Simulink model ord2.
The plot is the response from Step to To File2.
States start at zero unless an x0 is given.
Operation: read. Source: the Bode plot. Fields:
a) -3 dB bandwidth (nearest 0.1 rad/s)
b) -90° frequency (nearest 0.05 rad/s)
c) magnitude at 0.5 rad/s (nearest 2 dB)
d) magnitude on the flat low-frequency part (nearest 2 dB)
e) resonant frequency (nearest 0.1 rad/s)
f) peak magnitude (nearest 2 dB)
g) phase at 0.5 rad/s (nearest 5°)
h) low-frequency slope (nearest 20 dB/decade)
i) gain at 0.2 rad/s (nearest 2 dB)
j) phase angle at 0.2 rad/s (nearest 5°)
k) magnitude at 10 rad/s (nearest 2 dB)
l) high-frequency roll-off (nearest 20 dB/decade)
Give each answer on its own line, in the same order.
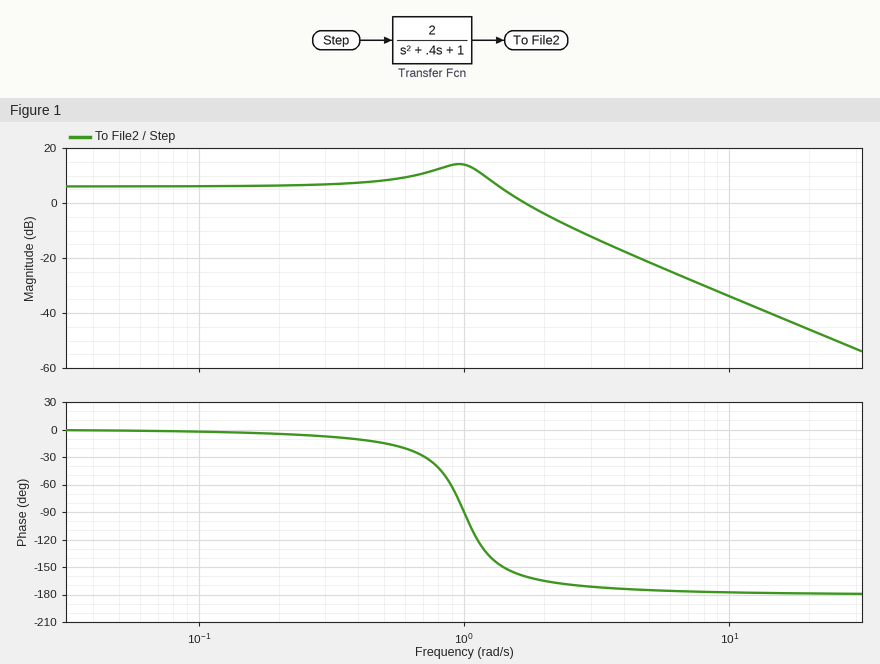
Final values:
1.5 rad/s
1.00 rad/s
8 dB
6 dB
1.0 rad/s
14 dB
-15°
0 dB/decade
6 dB
-5°
-34 dB
-40 dB/decade
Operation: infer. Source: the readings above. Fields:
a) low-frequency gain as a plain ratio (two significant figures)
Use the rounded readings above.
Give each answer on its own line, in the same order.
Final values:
2.0
